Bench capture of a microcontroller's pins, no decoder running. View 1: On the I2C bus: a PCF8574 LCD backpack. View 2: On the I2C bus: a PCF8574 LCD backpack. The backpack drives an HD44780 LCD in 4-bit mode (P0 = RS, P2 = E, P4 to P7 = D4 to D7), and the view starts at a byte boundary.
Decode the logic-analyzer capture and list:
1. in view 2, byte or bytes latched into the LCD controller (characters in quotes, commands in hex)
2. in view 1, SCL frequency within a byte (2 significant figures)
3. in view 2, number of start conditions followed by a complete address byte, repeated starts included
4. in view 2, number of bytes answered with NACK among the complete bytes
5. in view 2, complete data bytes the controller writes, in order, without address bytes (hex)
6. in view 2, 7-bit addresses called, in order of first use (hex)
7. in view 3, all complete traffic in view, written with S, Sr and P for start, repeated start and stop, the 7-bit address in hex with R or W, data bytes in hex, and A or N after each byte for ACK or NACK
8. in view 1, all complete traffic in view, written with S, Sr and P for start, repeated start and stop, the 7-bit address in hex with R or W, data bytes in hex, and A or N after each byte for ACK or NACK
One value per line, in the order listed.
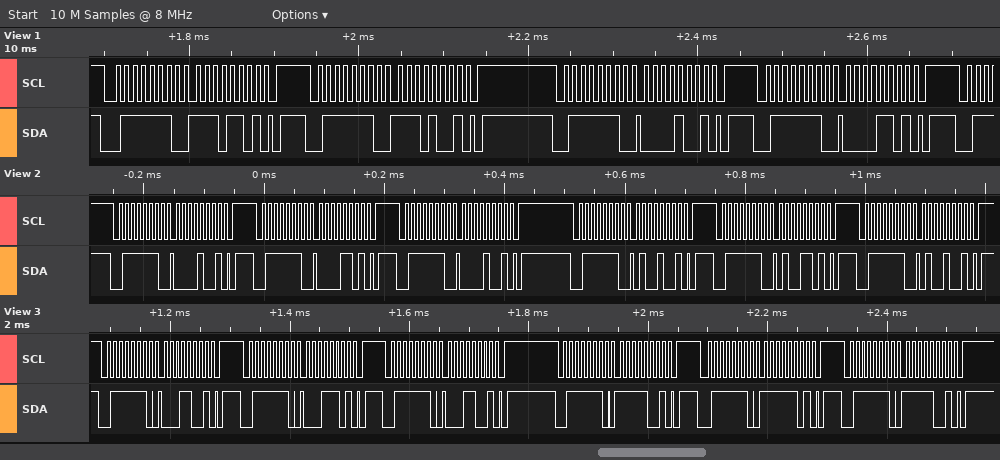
data 0x04
100 kHz
6
0
09 0D 09 49 4D 49
0x3F
S 3FW A 19 A P S 3FW A 1D A P S 3FW A 19 A P S 3FW A F9 A P S 3FW A FD A P S 3FW A F9 A P
S 3FW A ED A P S 3FW A E9 A P S 3FW A 09 A P S 3FW A 0D A P
